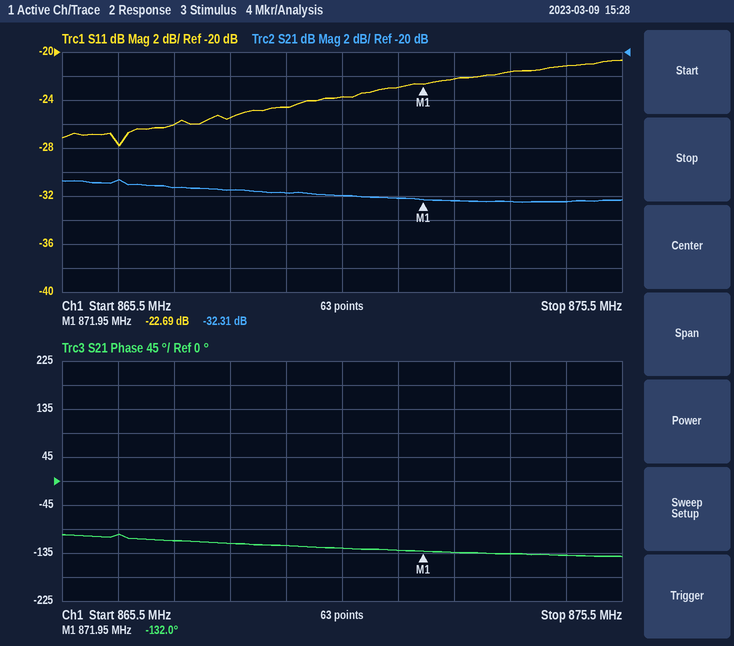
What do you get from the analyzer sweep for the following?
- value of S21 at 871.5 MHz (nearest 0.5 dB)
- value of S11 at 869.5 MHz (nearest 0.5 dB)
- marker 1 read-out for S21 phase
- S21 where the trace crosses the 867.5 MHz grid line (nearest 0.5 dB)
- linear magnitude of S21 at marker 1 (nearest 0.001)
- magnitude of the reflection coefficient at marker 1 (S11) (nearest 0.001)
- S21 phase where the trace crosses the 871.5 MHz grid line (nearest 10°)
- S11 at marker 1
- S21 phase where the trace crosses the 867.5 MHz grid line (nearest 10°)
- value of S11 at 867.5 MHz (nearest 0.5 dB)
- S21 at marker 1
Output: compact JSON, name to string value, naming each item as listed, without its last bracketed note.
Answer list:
{"value of S21 at 871.5 MHz": "-32.0 dB", "value of S11 at 869.5 MHz": "-24.5 dB", "marker 1 read-out for S21 phase": "-132.0°", "S21 where the trace crosses the 867.5 MHz grid line": "-31.5 dB", "linear magnitude of S21 at marker 1": "0.024", "magnitude of the reflection coefficient at marker 1 (S11)": "0.073", "S21 phase where the trace crosses the 871.5 MHz grid line": "-130°", "S11 at marker 1": "-22.69 dB", "S21 phase where the trace crosses the 867.5 MHz grid line": "-110°", "value of S11 at 867.5 MHz": "-26.0 dB", "S21 at marker 1": "-32.31 dB"}
